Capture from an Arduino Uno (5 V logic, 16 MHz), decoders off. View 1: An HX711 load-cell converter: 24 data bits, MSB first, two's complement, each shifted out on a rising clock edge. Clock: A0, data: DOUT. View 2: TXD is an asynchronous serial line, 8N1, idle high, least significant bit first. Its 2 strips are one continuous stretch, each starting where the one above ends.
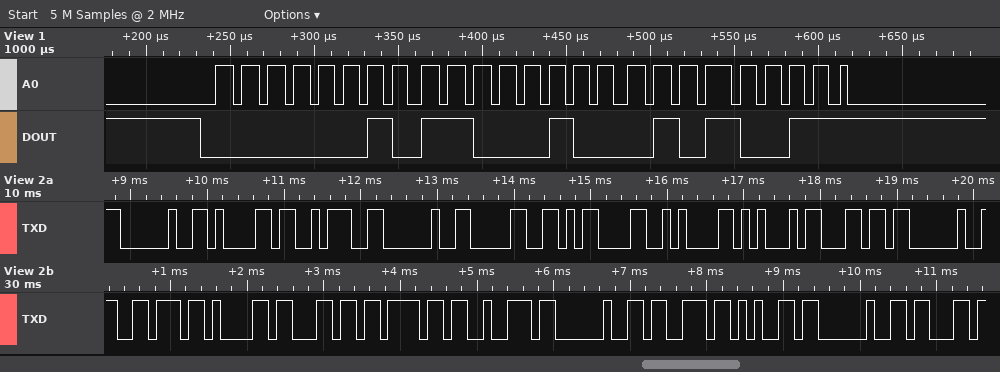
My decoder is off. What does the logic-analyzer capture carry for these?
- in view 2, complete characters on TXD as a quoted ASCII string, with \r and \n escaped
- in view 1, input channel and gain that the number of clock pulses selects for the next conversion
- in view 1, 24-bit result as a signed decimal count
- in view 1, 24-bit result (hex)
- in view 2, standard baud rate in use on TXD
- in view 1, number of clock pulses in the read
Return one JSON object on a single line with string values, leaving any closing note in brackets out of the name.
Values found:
{"in view 2, complete characters on TXD as a quoted ASCII string, with \\r and \\n escaped": "\" a: 0\\r\\nEl valor se c\"", "in view 1, input channel and gain that the number of clock pulses selects for the next conversion": "channel A, gain 128", "in view 1, 24-bit result as a signed decimal count": "181331", "in view 1, 24-bit result": "0x02C453", "in view 2, standard baud rate in use on TXD": "9600 baud", "in view 1, number of clock pulses in the read": "25"}
